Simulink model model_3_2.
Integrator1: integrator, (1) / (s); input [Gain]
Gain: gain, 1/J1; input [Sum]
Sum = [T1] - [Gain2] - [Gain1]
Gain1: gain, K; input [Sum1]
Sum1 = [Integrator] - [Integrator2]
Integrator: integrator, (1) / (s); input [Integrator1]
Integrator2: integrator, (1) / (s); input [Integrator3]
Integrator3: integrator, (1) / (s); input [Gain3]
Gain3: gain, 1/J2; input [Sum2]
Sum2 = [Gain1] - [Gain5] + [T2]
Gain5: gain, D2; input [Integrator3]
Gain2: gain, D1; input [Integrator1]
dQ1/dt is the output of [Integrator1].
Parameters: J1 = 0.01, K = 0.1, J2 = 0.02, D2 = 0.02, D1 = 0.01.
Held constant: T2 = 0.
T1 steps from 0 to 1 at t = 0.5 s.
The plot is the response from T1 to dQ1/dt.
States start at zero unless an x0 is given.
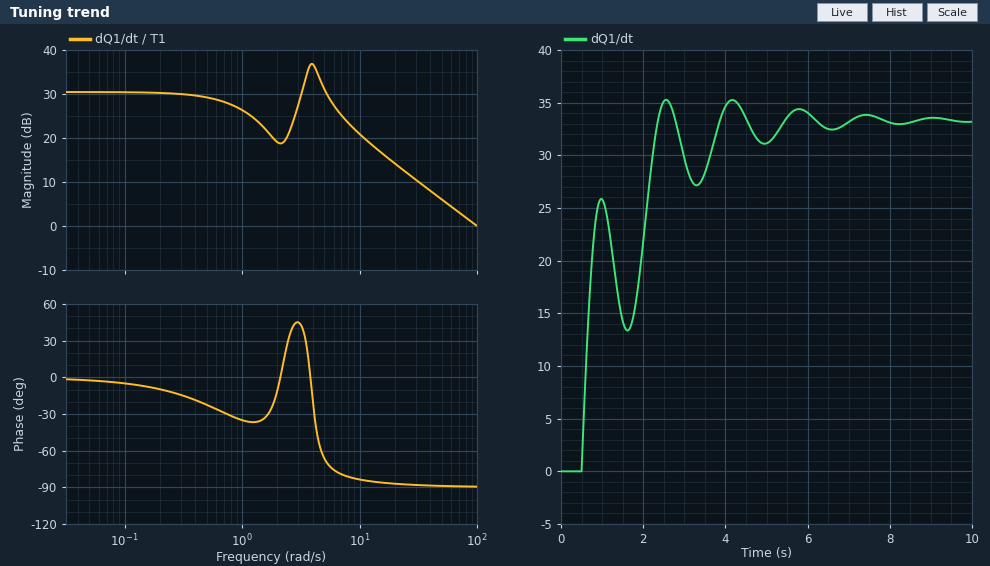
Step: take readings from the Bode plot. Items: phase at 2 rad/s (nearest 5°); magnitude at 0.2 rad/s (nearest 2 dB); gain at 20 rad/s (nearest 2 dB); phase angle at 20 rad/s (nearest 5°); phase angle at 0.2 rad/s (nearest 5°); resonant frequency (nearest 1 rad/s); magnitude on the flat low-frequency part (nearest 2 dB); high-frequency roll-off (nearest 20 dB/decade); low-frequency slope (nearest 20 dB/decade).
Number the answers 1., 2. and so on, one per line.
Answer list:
1. -10°
2. 30 dB
3. 14 dB
4. -85°
5. -10°
6. 4 rad/s
7. 30 dB
8. -20 dB/decade
9. 0 dB/decade
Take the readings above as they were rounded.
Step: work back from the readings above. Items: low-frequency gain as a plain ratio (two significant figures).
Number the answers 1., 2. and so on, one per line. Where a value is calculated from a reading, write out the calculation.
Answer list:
1. 10^(30 / 20) = 32
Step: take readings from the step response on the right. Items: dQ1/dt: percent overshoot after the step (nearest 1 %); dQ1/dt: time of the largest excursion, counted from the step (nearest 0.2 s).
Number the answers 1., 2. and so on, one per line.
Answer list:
1. 6 %
2. 2.0 s
